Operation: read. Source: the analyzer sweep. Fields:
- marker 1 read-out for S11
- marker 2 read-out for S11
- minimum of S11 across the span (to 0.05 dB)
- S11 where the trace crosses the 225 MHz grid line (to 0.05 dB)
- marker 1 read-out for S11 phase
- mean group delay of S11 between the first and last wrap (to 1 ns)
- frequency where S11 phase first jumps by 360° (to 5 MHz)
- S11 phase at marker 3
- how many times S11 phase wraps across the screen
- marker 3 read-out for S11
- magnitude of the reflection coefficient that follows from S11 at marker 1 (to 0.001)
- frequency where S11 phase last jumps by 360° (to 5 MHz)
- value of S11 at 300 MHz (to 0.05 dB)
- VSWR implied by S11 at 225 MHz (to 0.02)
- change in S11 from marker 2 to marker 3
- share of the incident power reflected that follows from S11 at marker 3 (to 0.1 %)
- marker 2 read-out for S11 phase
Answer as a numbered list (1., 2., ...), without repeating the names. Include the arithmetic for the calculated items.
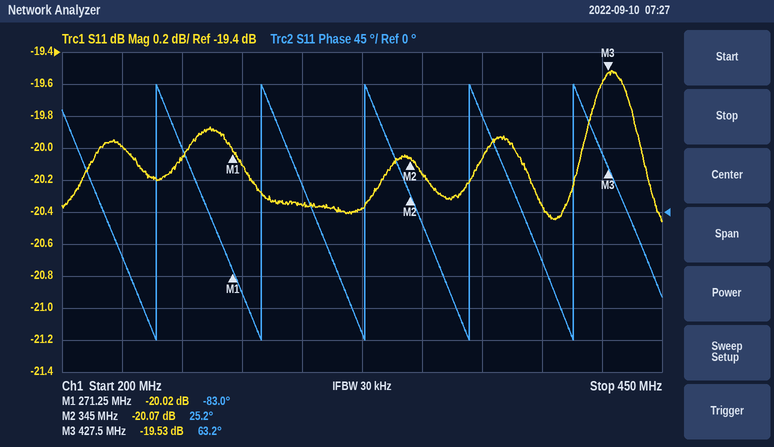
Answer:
1. -20.02 dB
2. -20.07 dB
3. -20.45 dB
4. -20.00 dB
5. -83.0°
6. 4 cycles / (415 MHz − 240 MHz) ≈ 23 ns
7. 240 MHz
8. 63.2°
9. 5
10. -19.53 dB
11. 10^(-20.02/20) ≈ 0.100
12. 415 MHz
13. -20.35 dB
14. |Γ| = 10^(-20/20) = 0.1000; VSWR = (1 + 0.1000)/(1 − 0.1000) ≈ 1.22
15. -19.53 − (-20.07) = 0.54 dB
16. 10^(-19.53/10) ≈ 1.1 %
17. 25.2°
